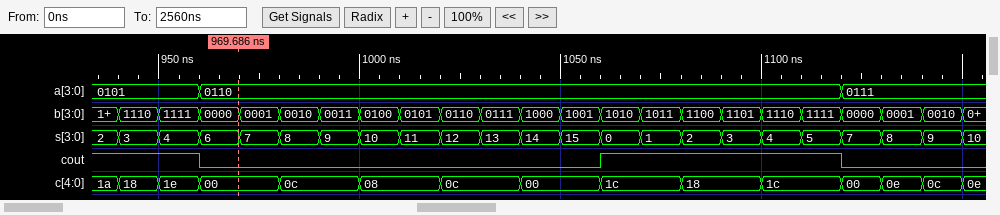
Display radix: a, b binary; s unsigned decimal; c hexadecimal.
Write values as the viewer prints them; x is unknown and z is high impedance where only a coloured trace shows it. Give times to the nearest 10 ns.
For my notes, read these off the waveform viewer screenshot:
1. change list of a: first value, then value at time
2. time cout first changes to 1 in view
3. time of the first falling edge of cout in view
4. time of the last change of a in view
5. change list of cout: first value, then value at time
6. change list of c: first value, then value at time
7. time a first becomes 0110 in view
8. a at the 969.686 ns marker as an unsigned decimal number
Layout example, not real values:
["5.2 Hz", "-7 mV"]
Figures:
["0101, 0110 at 960 ns, 0111 at 1120 ns", "1060 ns", "960 ns", "1120 ns", "1, 0 at 960 ns, 1 at 1060 ns, 0 at 1120 ns", "1a, 18 at 940 ns, 1e at 950 ns, 00 at 960 ns, 0c at 980 ns, 08 at 1000 ns, 0c at 1020 ns, 00 at 1040 ns, 1c at 1060 ns, 18 at 1080 ns, 1c at 1100 ns, 00 at 1120 ns, 0e at 1130 ns, 0c at 1140 ns, 0e at 1150 ns", "960 ns", "6"]
